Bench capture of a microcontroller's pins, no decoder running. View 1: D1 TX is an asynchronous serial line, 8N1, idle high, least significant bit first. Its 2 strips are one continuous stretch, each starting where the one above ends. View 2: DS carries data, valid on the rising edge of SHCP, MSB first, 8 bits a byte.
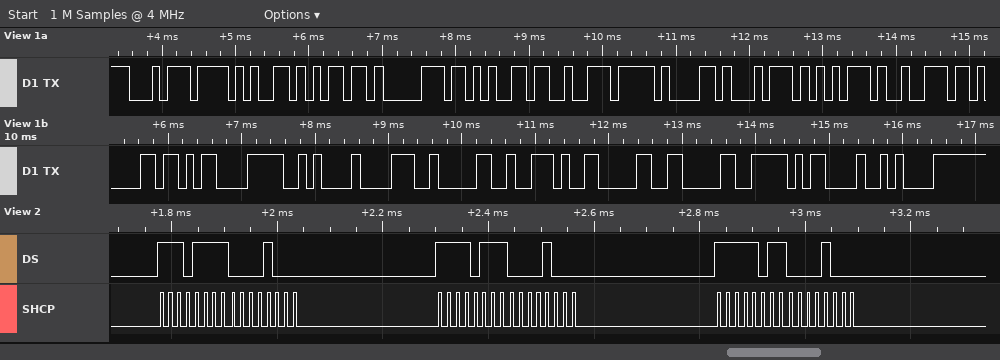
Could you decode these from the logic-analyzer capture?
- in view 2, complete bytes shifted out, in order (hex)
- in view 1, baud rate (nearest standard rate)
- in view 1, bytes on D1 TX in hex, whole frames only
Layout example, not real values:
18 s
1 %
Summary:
EF 08 F7 08 FB 08
9600 baud
0x74 0x65 0x6D 0x70 0x65 0x72 0x61 0x74 0x75 0x72 0x61 0x0D 0x0A 0x38 0x30 0x2E 0x30 0x30 0x0D 0x0A
